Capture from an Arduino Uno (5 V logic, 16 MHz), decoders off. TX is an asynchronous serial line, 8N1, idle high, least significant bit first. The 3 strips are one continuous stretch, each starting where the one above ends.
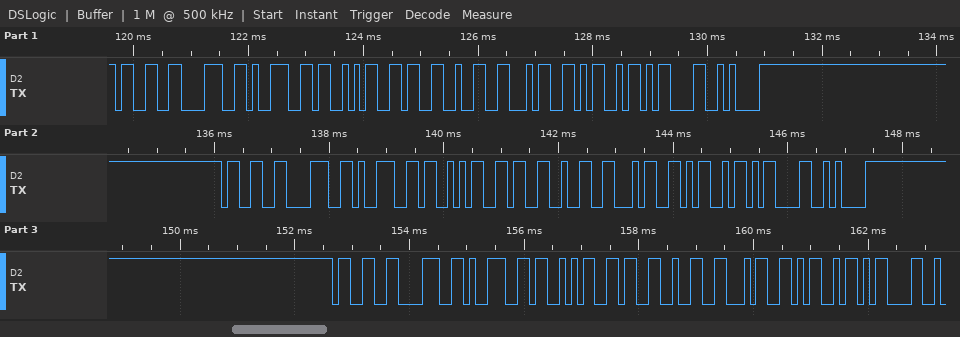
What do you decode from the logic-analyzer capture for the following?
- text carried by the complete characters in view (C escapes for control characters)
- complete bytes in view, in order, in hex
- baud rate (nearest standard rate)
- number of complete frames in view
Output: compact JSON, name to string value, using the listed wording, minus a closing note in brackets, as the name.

{"text carried by the complete characters in view": "\"389S624M\\r\\n389S624M\\r\\n389S624M\\r\"", "complete bytes in view, in order, in hex": "0x33 0x38 0x39 0x53 0x36 0x32 0x34 0x4D 0x0D 0x0A 0x33 0x38 0x39 0x53 0x36 0x32 0x34 0x4D 0x0D 0x0A 0x33 0x38 0x39 0x53 0x36 0x32 0x34 0x4D 0x0D", "baud rate": "9600 baud", "number of complete frames in view": "29"}
